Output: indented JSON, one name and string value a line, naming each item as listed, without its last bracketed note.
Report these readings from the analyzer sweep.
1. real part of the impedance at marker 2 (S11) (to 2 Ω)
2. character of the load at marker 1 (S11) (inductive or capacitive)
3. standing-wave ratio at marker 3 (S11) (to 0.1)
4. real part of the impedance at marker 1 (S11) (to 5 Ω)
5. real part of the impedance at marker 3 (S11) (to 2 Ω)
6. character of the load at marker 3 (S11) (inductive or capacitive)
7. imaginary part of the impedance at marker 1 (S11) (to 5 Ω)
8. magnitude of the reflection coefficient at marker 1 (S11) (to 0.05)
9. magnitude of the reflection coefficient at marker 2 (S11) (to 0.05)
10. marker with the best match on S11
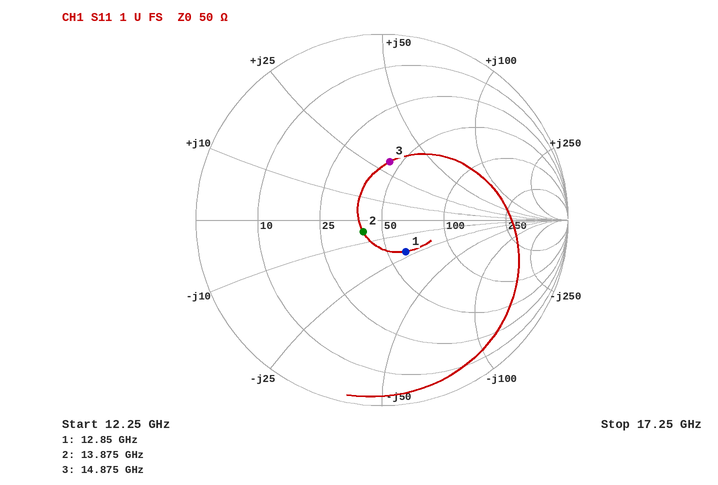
{
  "real part of the impedance at marker 2 (S11)": "40 Ω",
  "character of the load at marker 1 (S11)": "capacitive",
  "standing-wave ratio at marker 3 (S11)": "1.9",
  "real part of the impedance at marker 1 (S11)": "60 Ω",
  "real part of the impedance at marker 3 (S11)": "44 Ω",
  "character of the load at marker 3 (S11)": "inductive",
  "imaginary part of the impedance at marker 1 (S11)": "-20 Ω",
  "magnitude of the reflection coefficient at marker 1 (S11)": "0.20",
  "magnitude of the reflection coefficient at marker 2 (S11)": "0.10",
  "marker with the best match on S11": "marker 2"
}
